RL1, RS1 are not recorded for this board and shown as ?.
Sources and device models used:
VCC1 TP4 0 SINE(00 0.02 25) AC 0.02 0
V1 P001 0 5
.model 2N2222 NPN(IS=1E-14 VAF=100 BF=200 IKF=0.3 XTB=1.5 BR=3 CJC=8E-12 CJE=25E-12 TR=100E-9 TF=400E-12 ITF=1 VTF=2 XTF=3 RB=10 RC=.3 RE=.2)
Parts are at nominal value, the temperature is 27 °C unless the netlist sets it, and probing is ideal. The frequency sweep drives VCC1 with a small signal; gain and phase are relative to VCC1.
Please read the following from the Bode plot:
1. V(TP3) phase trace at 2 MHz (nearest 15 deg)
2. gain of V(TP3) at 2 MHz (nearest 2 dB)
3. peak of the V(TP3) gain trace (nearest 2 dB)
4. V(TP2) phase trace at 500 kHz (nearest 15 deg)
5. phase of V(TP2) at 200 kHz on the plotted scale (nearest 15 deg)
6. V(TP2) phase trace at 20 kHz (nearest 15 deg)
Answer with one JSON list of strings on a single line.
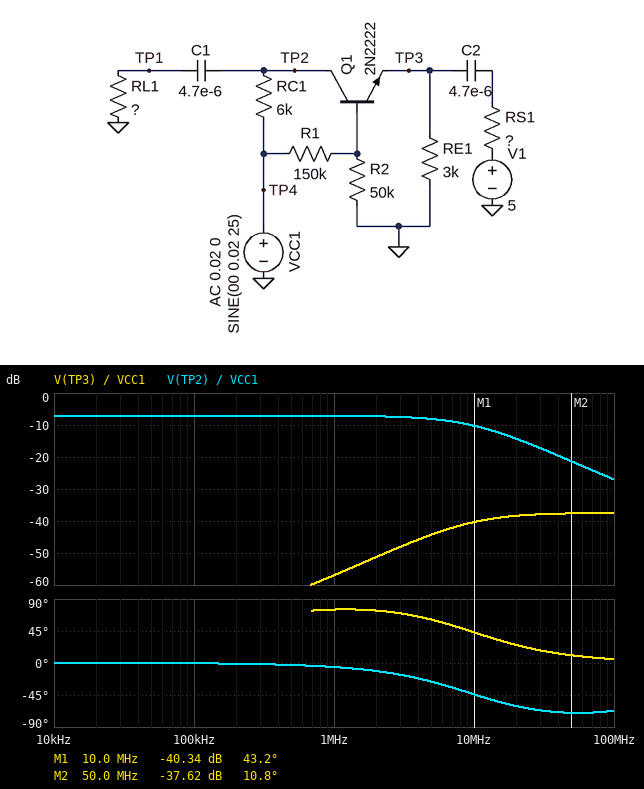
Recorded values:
["75 deg", "-52 dB", "-38 dB", "0 deg", "0 deg", "0 deg"]
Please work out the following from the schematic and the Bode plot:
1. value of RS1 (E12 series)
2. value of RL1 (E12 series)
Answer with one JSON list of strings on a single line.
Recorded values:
["82 Ω", "4.7 kΩ"]
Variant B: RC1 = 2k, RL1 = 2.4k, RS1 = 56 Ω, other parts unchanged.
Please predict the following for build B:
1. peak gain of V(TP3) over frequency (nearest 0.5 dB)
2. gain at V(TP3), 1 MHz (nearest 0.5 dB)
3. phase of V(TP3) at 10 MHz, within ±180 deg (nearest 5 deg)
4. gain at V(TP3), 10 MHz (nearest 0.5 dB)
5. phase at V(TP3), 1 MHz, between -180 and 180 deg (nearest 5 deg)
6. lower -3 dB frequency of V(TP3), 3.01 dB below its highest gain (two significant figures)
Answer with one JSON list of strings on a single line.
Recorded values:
["-31.5 dB", "-58.5 dB", "65 deg", "-39.5 dB", "80 deg", "23 MHz"]
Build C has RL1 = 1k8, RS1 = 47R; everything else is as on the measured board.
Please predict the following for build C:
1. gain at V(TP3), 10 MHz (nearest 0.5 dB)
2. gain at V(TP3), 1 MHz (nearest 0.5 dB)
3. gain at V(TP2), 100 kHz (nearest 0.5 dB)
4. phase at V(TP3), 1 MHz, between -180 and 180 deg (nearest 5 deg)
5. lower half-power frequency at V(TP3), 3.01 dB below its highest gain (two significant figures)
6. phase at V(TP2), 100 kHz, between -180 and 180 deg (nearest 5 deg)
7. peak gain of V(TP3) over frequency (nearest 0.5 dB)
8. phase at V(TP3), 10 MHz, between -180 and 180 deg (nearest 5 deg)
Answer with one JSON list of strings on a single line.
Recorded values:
["-48.5 dB", "-66.5 dB", "-12.5 dB", "65 deg", "18 MHz", "0 deg", "-42.0 dB", "60 deg"]
